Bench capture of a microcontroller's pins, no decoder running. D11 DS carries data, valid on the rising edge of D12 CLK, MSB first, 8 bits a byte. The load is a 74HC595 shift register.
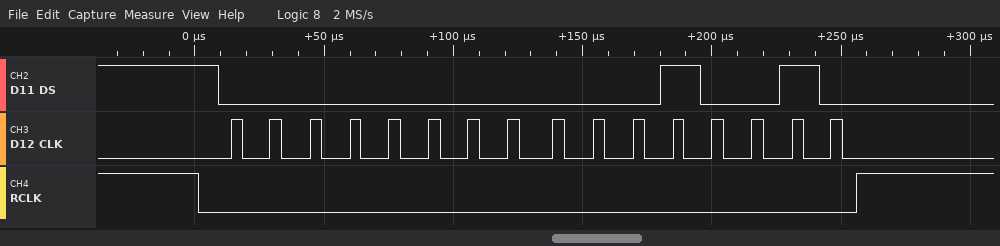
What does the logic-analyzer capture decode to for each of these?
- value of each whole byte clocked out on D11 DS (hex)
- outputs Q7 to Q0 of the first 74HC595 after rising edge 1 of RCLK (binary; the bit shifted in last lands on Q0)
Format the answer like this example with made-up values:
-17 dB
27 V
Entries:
00 12
00010010
